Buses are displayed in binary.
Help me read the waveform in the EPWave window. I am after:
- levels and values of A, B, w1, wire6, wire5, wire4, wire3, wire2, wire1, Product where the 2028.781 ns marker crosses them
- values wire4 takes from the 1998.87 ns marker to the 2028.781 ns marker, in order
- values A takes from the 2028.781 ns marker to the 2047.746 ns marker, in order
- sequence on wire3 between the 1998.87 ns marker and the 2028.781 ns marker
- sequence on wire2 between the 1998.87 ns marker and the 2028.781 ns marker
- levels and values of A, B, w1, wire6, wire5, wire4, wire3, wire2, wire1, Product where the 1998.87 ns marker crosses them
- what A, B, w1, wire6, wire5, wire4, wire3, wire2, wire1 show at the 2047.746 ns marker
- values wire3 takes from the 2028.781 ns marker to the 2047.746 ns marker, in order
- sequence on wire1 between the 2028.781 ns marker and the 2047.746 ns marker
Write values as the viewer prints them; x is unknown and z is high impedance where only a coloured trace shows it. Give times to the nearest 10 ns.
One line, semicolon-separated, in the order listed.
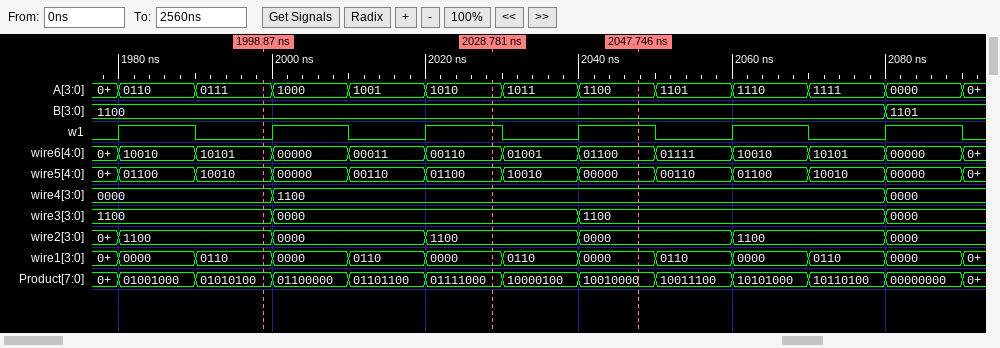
A=1010, B=1100, w1=1, wire6=00110, wire5=01100, wire4=1100, wire3=0000, wire2=1100, wire1=0000, Product=01111000; 0000, 1100; 1010, 1011, 1100; 1100, 0000; 1100, 0000, 1100; A=0111, B=1100, w1=0, wire6=10101, wire5=10010, wire4=0000, wire3=1100, wire2=1100, wire1=0110, Product=01010100; A=1100, B=1100, w1=1, wire6=01100, wire5=00000, wire4=1100, wire3=1100, wire2=0000, wire1=0000; 0000, 1100; 0000, 0110, 0000
